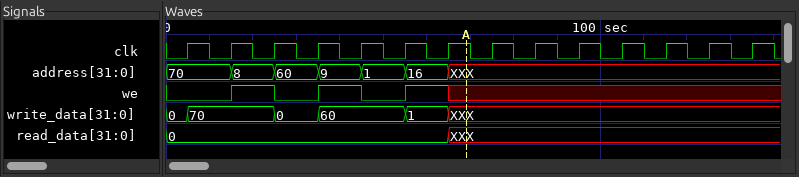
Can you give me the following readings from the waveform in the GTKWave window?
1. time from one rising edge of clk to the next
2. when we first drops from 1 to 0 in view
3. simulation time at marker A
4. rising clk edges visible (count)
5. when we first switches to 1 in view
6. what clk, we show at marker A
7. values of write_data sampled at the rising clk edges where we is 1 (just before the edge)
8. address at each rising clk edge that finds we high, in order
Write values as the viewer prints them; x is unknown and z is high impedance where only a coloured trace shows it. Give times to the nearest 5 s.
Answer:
10 s
25 s
70 s
14
15 s
clk=1, we=x
70, 60, 1
8, 9, 16
